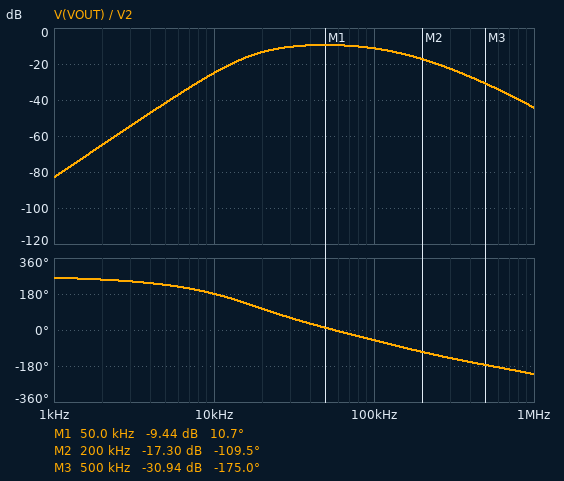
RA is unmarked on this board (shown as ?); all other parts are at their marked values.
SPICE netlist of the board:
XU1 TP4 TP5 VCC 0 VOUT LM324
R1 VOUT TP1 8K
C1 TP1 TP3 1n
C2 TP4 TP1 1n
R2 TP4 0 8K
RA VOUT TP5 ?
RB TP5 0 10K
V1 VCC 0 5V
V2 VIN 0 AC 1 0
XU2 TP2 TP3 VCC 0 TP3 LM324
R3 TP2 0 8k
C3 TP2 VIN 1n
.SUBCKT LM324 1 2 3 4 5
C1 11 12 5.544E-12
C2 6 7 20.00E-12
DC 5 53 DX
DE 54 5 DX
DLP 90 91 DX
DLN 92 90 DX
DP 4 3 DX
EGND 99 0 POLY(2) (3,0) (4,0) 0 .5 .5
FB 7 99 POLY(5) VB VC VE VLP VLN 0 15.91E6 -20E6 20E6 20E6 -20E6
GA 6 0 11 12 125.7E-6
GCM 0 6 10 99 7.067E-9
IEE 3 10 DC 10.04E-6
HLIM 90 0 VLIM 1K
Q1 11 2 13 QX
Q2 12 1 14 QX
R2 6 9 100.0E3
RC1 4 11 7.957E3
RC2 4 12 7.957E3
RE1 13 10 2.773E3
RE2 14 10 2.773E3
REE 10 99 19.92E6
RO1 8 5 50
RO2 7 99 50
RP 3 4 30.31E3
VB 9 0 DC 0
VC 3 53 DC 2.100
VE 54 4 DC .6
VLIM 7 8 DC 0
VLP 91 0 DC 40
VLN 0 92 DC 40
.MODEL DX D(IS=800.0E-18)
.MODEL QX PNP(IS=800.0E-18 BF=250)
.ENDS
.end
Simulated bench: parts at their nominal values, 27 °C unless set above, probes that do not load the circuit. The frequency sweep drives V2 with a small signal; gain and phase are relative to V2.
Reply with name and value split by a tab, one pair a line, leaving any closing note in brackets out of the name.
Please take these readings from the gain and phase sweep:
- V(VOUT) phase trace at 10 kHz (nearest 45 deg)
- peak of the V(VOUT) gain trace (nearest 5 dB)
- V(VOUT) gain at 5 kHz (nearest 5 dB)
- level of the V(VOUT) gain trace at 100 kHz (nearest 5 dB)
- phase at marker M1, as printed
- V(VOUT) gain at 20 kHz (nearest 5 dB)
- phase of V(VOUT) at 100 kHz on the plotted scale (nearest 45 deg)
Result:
V(VOUT) phase trace at 10 kHz	180 deg
peak of the V(VOUT) gain trace	-10 dB
V(VOUT) gain at 5 kHz	-40 dB
level of the V(VOUT) gain trace at 100 kHz	-10 dB
phase at marker M1, as printed	10.7 deg
V(VOUT) gain at 20 kHz	-15 dB
phase of V(VOUT) at 100 kHz on the plotted scale	-45 deg
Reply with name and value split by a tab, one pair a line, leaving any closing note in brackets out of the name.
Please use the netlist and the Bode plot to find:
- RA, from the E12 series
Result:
RA, from the E12 series	27 kΩ
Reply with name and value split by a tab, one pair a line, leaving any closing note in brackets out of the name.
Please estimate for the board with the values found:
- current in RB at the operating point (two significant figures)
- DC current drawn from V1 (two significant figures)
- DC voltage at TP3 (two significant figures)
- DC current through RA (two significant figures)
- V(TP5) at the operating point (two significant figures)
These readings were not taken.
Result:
current in RB at the operating point	1.4 µA
DC current drawn from V1	350 µA
DC voltage at TP3	30 mV
DC current through RA	1.4 µA
V(TP5) at the operating point	14 mV
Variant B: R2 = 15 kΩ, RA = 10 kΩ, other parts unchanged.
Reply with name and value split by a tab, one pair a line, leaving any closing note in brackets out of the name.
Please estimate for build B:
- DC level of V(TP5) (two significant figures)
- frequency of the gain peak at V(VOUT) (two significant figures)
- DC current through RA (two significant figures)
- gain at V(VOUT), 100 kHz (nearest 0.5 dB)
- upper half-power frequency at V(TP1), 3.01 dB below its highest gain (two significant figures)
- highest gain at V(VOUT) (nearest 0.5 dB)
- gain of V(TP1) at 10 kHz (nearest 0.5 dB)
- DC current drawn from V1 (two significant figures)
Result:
DC level of V(TP5)	20 mV
frequency of the gain peak at V(VOUT)	48 kHz
DC current through RA	2.0 µA
gain at V(VOUT), 100 kHz	-14.5 dB
upper half-power frequency at V(TP1), 3.01 dB below its highest gain	200 kHz
highest gain at V(VOUT)	-12.5 dB
gain of V(TP1) at 10 kHz	-19.5 dB
DC current drawn from V1	350 µA
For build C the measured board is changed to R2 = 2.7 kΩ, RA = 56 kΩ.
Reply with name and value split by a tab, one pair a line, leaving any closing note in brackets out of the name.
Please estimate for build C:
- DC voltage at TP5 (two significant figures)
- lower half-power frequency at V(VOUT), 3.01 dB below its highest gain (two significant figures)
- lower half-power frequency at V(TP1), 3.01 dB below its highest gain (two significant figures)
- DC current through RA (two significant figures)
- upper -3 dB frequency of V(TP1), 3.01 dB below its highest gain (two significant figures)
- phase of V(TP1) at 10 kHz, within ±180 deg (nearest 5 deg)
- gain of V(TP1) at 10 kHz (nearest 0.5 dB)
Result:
DC voltage at TP5	9.3 mV
lower half-power frequency at V(VOUT), 3.01 dB below its highest gain	33 kHz
lower half-power frequency at V(TP1), 3.01 dB below its highest gain	20 kHz
DC current through RA	910 nA
upper -3 dB frequency of V(TP1), 3.01 dB below its highest gain	260 kHz
phase of V(TP1) at 10 kHz, within ±180 deg	115 deg
gain of V(TP1) at 10 kHz	-21.5 dB
